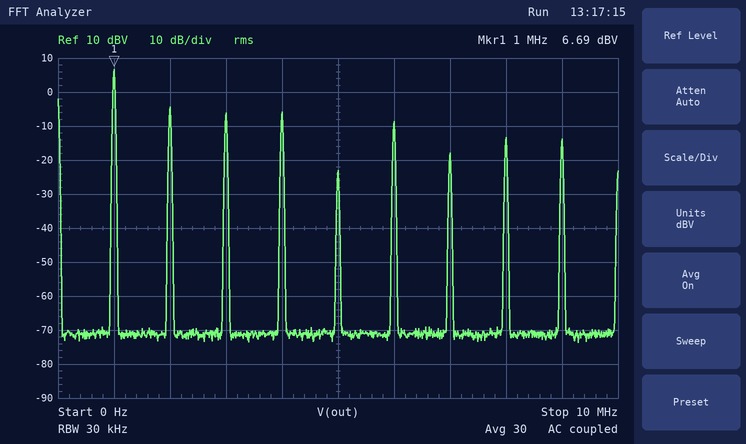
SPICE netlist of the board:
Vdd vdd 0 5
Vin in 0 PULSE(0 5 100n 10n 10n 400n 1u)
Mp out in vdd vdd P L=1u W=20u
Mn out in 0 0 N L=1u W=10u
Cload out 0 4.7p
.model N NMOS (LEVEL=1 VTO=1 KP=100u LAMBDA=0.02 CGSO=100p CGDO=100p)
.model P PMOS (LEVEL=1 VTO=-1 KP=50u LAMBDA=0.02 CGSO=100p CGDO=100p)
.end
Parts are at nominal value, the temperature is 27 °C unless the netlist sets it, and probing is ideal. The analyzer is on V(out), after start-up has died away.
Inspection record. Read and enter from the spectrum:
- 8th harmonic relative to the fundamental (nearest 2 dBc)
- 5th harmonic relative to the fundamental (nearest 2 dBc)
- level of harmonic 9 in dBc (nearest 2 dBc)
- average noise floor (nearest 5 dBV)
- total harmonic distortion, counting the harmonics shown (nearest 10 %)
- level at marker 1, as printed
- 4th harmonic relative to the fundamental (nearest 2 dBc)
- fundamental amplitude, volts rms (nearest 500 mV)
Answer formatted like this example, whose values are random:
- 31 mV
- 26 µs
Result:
- -20 dBc
- -30 dBc
- -20 dBc
- -70 dBV
- 50 %
- 6.69 dBV
- -12 dBc
- 2.0 V
